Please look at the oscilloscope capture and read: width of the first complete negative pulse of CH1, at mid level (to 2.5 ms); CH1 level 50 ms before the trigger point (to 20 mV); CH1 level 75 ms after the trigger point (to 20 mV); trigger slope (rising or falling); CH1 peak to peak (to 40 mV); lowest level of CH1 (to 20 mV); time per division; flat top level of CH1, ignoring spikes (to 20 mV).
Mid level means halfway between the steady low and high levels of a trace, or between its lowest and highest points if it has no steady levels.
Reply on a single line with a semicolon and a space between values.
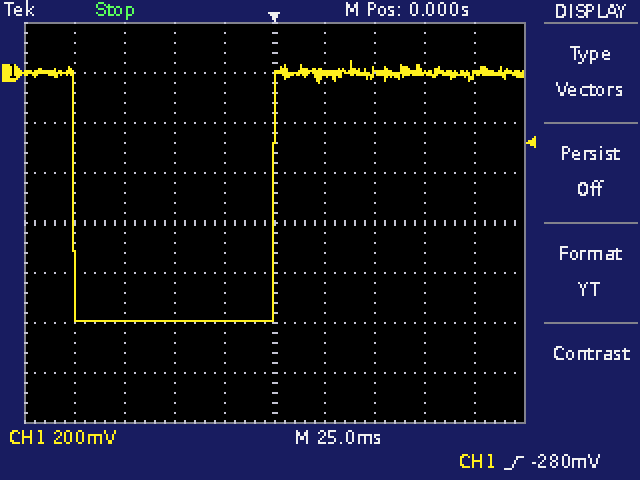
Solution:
100.0 ms; -1.00 V; 0 mV; rising; 1.04 V; -1.00 V; 25 ms; 0 mV
